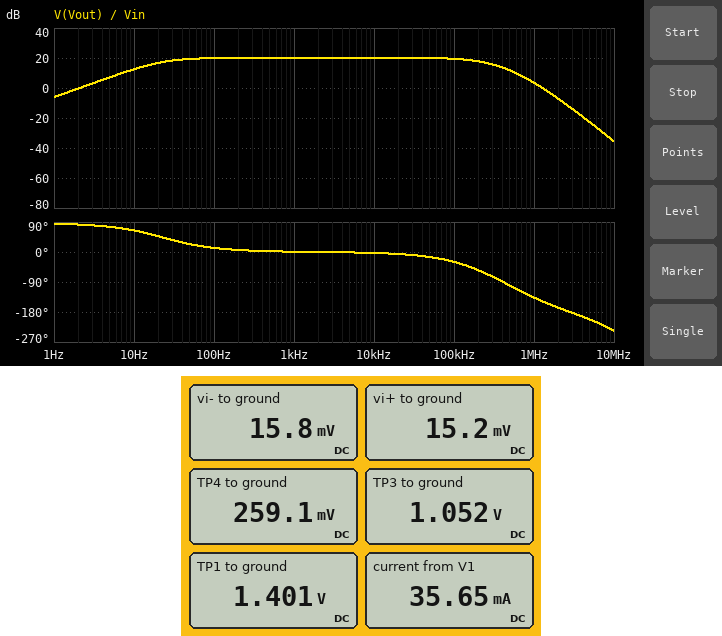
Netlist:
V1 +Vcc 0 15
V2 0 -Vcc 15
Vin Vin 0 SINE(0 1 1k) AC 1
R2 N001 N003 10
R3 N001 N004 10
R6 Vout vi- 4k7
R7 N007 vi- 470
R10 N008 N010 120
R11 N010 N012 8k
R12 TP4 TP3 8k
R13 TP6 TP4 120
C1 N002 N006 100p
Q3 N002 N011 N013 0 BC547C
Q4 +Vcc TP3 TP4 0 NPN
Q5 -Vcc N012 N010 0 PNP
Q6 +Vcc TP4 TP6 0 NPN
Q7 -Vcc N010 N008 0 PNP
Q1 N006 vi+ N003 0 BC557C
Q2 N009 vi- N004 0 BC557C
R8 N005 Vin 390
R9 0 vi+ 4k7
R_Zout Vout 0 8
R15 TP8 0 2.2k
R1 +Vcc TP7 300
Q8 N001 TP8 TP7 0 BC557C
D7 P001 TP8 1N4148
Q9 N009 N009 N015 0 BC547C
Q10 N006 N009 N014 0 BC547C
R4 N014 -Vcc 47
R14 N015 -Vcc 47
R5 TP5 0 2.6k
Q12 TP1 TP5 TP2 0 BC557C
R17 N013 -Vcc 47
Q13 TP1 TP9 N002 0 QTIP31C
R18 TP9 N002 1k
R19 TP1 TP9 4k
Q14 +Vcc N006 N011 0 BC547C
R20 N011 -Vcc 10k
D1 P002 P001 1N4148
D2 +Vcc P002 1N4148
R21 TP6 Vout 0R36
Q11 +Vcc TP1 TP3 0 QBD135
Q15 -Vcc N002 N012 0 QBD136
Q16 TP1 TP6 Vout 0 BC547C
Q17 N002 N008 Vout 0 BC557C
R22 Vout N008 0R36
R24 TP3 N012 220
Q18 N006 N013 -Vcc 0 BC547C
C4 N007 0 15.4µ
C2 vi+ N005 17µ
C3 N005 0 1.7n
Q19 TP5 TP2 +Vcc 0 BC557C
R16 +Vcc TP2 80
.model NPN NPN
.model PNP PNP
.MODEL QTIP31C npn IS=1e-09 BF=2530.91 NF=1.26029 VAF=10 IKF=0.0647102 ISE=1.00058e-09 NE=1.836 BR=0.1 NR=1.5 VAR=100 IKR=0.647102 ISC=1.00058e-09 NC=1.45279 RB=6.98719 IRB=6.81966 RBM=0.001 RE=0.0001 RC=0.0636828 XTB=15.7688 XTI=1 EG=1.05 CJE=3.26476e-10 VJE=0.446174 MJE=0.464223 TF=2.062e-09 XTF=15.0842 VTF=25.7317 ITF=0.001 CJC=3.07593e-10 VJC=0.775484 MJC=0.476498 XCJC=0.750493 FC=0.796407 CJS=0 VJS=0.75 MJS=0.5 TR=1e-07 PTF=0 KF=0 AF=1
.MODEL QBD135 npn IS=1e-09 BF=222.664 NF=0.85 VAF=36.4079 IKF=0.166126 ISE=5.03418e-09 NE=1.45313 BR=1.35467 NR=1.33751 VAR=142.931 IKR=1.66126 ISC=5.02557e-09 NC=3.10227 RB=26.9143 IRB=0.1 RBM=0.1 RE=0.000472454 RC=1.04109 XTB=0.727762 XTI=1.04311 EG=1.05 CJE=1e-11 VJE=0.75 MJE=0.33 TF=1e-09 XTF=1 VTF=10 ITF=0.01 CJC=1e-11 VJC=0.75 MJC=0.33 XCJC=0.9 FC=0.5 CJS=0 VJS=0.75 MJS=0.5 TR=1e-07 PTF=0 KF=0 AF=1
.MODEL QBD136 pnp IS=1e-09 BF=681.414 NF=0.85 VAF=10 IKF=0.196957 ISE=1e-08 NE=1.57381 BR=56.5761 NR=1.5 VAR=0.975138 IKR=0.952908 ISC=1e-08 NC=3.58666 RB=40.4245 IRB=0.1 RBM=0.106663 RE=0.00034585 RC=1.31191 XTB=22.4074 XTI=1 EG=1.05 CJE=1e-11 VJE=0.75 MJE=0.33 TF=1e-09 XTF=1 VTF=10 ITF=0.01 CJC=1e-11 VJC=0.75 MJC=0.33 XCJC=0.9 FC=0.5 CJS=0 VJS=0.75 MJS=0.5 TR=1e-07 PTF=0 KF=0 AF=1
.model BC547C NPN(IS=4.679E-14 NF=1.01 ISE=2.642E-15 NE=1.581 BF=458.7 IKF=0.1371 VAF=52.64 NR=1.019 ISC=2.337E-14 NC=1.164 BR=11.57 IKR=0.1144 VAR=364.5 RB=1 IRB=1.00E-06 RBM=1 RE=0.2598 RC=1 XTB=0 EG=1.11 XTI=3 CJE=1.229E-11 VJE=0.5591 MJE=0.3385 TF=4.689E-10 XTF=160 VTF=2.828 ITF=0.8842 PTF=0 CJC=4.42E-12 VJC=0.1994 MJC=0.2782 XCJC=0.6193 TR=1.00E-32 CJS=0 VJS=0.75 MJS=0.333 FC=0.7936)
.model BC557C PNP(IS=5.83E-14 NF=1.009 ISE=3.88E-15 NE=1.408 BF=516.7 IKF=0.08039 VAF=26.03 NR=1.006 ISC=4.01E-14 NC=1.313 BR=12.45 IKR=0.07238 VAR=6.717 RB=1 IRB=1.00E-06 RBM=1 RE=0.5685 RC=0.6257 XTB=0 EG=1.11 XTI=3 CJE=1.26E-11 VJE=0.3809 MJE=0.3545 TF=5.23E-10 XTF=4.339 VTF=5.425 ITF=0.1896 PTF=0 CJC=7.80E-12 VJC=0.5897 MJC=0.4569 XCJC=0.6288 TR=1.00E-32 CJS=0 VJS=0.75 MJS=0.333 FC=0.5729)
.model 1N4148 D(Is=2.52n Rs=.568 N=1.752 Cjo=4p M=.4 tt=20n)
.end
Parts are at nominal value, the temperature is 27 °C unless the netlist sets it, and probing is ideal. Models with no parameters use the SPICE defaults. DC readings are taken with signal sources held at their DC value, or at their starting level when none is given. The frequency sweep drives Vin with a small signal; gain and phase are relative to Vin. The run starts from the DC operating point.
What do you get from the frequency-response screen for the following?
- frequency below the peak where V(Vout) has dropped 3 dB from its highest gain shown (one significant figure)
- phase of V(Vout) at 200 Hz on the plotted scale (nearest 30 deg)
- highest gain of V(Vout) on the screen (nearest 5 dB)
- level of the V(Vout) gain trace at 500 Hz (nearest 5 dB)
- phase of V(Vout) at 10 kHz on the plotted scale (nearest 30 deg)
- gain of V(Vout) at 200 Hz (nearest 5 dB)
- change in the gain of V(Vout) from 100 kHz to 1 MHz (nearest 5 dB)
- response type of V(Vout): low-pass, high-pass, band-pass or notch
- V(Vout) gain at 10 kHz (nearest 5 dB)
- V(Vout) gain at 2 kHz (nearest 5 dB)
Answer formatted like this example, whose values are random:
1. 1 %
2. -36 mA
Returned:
1. 20 Hz
2. 0 deg
3. 20 dB
4. 20 dB
5. 0 deg
6. 20 dB
7. -15 dB
8. band-pass
9. 20 dB
10. 20 dB
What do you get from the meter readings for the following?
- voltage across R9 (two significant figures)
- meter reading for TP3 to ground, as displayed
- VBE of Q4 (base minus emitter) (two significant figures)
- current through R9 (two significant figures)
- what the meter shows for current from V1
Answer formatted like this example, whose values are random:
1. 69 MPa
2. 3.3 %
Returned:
1. 15 mV
2. 1.052 V
3. 790 mV
4. 3.2 µA
5. 35.65 mA
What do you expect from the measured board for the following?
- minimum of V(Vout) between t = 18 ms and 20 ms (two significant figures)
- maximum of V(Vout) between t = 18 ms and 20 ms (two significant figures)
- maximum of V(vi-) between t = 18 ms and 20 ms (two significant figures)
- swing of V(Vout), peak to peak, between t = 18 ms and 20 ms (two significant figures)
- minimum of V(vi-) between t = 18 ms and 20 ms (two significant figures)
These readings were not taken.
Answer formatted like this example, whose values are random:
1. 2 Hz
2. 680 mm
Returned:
1. -10 V
2. 10 V
3. 940 mV
4. 20 V
5. -910 mV
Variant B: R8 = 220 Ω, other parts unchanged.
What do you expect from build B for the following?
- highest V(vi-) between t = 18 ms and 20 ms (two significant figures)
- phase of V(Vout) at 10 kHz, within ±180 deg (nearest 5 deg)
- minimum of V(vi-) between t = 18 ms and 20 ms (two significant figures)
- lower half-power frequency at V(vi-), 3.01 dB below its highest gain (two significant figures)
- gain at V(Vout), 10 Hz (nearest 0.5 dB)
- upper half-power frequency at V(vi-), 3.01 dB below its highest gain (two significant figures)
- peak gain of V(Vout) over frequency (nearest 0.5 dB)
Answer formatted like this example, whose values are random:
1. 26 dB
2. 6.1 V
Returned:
1. 970 mV
2. 0 deg
3. -940 mV
4. 1.9 Hz
5. 13.0 dB
6. 350 kHz
7. 20.5 dB
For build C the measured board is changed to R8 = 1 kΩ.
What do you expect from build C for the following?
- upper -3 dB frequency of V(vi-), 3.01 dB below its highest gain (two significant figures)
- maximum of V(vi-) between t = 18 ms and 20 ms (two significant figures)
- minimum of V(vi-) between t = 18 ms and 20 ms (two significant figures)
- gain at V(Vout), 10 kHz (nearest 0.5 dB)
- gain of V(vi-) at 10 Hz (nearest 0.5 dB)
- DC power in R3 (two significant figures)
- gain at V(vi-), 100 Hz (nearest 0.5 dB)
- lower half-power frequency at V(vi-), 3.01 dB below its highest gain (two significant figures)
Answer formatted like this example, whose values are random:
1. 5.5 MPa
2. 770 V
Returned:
1. 110 kHz
2. 840 mV
3. -810 mV
4. 19.0 dB
5. -2.0 dB
6. 51 µW
7. -1.5 dB
8. 1.6 Hz
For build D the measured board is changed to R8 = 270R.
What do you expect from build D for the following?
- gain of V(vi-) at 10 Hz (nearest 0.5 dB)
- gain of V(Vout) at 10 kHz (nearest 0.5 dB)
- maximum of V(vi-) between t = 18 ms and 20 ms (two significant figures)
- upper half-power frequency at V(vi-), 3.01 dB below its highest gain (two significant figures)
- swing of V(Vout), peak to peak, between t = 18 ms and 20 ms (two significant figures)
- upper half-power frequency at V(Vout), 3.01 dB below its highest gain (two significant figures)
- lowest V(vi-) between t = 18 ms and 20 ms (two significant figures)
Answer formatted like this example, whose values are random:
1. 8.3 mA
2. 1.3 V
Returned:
1. -0.5 dB
2. 20.5 dB
3. 960 mV
4. 300 kHz
5. 21 V
6. 310 kHz
7. -930 mV
